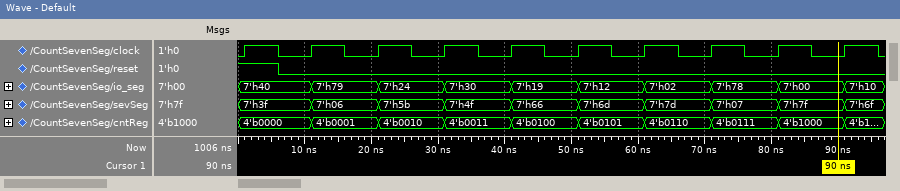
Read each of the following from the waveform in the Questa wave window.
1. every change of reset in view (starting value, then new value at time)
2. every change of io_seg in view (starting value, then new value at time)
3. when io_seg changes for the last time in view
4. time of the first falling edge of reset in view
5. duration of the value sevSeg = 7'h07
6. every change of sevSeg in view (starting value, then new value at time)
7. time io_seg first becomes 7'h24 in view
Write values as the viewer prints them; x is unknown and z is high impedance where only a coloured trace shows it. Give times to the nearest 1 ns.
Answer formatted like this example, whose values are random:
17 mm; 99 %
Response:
1, 0 at 6 ns; 7'h40, 7'h79 at 11 ns, 7'h24 at 21 ns, 7'h30 at 31 ns, 7'h19 at 41 ns, 7'h12 at 51 ns, 7'h02 at 61 ns, 7'h78 at 71 ns, 7'h00 at 81 ns, 7'h10 at 91 ns; 91 ns; 6 ns; 10 ns; 7'h3f, 7'h06 at 11 ns, 7'h5b at 21 ns, 7'h4f at 31 ns, 7'h66 at 41 ns, 7'h6d at 51 ns, 7'h7d at 61 ns, 7'h07 at 71 ns, 7'h7f at 81 ns, 7'h6f at 91 ns; 21 ns
